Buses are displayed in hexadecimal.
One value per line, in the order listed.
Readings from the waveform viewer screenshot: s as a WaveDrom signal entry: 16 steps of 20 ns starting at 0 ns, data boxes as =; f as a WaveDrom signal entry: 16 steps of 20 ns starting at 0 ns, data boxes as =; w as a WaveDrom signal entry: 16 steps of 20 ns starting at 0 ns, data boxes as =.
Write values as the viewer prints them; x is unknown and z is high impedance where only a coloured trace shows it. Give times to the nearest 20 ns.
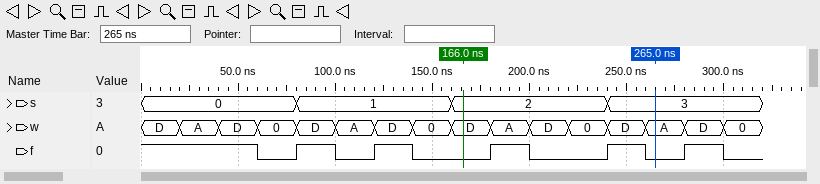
{name: 's', wave: '=...=...=...=...', data: '0 1 2 3'}
{name: 'f', wave: '1..01010.10.1010'}
{name: 'w', wave: '================', data: 'D A D 0 D A D 0 D A D 0 D A D 0'}
